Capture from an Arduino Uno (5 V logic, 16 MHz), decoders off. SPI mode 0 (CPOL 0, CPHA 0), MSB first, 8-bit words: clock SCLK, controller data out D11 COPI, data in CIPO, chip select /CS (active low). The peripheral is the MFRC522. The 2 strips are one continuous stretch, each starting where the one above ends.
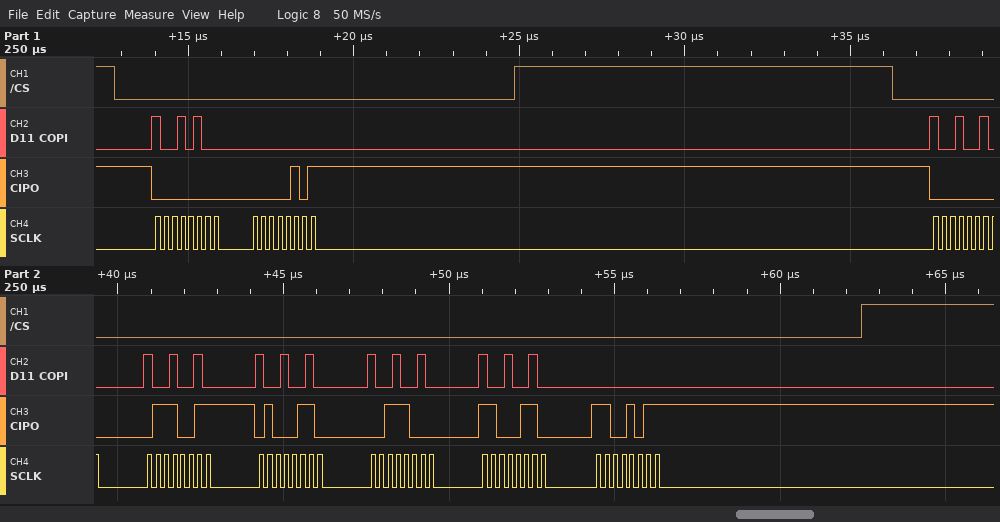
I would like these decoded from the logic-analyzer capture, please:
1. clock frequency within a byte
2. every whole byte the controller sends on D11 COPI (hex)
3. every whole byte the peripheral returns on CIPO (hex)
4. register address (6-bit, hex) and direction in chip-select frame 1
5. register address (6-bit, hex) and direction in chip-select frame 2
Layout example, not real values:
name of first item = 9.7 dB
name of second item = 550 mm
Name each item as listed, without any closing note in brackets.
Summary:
clock frequency within a byte = 4 MHz
every whole byte the controller sends on D11 COPI = 94 00 92 92 92 92 92 00
every whole byte the peripheral returns on CIPO = 00 05 00 73 46 38 C6 CB
register address (6-bit, hex) and direction in chip-select frame 1 = 0x0A read
register address (6-bit, hex) and direction in chip-select frame 2 = 0x09 read
